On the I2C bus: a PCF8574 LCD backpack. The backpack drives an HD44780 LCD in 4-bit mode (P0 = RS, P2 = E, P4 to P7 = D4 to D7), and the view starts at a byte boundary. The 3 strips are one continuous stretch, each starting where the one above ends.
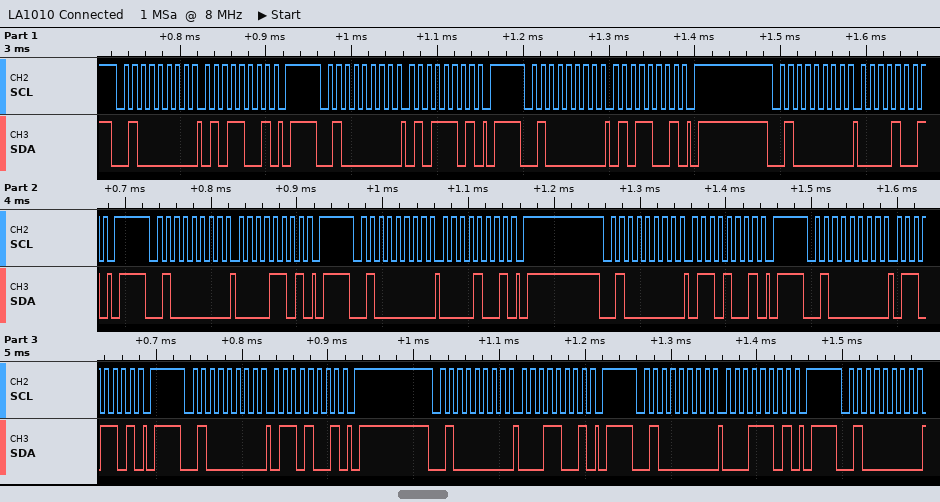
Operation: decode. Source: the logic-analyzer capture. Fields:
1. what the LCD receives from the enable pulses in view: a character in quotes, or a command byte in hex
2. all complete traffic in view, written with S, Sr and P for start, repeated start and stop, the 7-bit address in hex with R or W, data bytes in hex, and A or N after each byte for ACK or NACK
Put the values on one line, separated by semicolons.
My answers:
'P'; S 20W A 59 A P S 20W A 5D A P S 20W A 59 A P S 20W A 09 A P S 20W A 0D A P S 20W A 09 A P S 20W A 69 A P S 20W A 6D A P S 20W A 69 A P S 20W A 19 A P S 20W A 1D A P S 20W A
